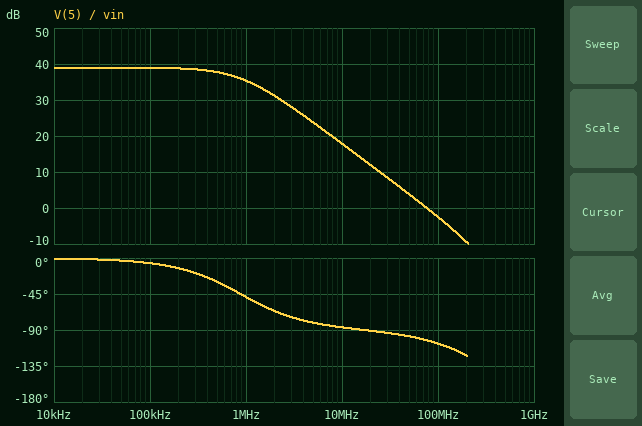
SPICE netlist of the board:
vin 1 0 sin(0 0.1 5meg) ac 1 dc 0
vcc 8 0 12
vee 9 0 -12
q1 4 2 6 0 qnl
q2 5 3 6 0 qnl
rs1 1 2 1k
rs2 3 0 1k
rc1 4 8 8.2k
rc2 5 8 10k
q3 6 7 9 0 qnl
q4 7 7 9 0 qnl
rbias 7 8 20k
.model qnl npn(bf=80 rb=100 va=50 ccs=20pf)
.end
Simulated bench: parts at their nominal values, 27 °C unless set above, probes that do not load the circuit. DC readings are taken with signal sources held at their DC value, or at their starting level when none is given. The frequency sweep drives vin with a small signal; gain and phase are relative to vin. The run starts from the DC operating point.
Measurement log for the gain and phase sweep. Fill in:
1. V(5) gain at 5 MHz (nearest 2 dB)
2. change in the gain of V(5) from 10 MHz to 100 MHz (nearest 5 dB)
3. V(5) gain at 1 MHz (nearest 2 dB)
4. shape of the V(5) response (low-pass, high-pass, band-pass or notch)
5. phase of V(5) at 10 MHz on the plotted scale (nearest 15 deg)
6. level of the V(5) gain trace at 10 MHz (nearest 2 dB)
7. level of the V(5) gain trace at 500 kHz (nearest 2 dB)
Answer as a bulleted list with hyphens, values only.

- 24 dB
- -20 dB
- 36 dB
- low-pass
- -90 deg
- 18 dB
- 38 dB
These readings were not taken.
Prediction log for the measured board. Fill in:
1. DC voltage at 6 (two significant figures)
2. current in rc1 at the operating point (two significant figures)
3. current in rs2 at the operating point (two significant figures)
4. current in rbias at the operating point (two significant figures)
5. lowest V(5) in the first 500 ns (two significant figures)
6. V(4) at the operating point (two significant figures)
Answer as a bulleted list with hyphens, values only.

- -770 mV
- 680 µA
- 7.6 µA
- 1.2 mA
- 4.3 V
- 6.4 V
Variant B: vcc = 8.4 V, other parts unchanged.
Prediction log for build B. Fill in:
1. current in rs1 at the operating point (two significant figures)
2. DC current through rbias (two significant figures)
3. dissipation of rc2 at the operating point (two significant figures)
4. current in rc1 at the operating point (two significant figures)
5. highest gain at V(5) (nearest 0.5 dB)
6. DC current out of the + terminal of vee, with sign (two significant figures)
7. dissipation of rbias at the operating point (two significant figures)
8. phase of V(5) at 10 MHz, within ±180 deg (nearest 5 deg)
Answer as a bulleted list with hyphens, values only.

- 6.7 µA
- 980 µA
- 3.2 mW
- 580 µA
- 38.0 dB
- -2.1 mA
- 19 mW
- -85 deg
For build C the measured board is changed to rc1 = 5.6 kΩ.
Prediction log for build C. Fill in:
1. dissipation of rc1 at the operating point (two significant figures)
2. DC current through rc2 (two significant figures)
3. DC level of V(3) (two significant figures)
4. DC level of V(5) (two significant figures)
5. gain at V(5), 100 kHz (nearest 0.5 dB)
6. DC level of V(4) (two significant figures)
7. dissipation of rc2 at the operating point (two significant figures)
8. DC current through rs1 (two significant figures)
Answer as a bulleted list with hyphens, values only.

- 2.7 mW
- 660 µA
- -7.5 mV
- 5.4 V
- 39.0 dB
- 8.1 V
- 4.4 mW
- 7.5 µA
